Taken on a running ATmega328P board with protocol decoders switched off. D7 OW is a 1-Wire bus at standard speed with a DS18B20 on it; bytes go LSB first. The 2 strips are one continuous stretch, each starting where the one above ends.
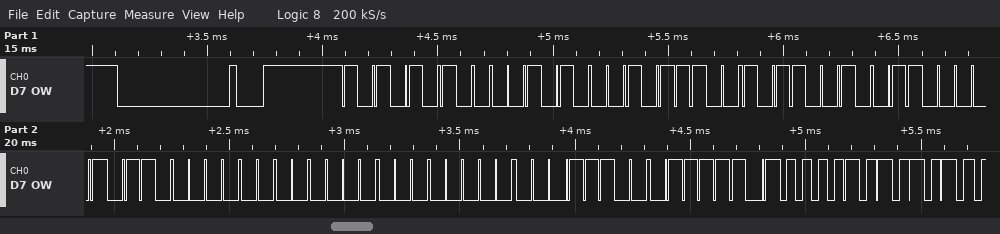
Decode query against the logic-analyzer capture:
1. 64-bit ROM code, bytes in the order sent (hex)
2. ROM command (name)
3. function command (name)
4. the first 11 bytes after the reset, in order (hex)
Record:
28 3A 4D 86 06 00 00 38
Match ROM
Read Scratchpad
55 28 3A 4D 86 06 00 00 38 BE 50
